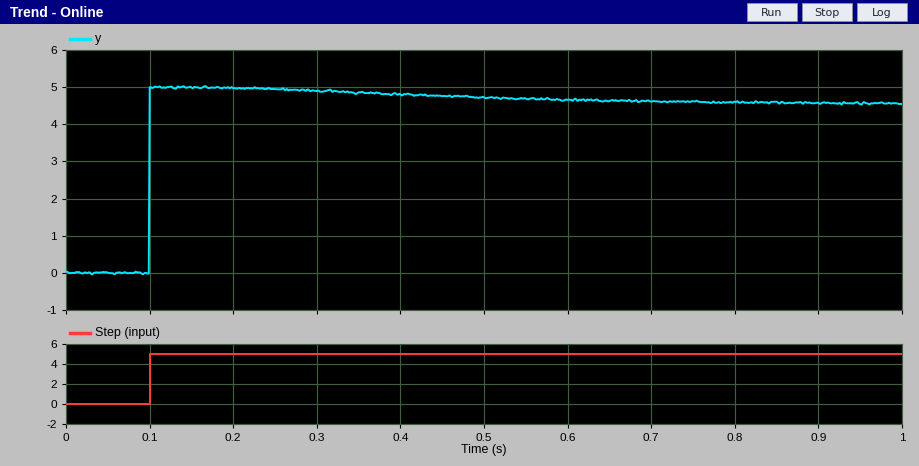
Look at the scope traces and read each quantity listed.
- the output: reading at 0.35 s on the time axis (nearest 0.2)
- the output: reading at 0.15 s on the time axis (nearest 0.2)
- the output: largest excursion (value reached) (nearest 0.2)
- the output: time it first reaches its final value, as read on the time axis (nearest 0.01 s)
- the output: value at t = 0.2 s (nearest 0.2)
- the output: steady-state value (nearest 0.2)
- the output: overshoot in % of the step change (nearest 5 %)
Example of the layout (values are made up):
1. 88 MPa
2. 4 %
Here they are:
1. 4.8
2. 5.0
3. 5.0
4. 0.10 s
5. 5.0
6. 4.6
7. 10 %
